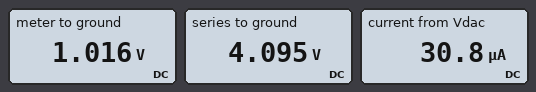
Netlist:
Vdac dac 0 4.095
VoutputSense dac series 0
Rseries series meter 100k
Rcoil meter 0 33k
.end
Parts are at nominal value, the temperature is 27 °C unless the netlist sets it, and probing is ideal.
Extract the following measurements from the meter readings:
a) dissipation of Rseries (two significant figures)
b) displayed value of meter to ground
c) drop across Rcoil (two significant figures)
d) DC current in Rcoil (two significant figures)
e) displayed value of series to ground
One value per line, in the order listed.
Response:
95 µW
1.016 V
1.0 V
31 µA
4.095 V
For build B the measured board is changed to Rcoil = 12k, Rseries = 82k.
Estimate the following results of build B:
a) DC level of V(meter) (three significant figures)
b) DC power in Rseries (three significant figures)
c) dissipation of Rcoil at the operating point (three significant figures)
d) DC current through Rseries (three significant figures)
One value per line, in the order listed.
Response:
523 mV
156 µW
22.8 µW
43.6 µA
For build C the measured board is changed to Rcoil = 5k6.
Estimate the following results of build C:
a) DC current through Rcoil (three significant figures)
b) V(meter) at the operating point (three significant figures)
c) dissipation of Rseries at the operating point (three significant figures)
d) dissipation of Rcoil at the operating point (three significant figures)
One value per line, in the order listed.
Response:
38.8 µA
217 mV
150 µW
8.42 µW
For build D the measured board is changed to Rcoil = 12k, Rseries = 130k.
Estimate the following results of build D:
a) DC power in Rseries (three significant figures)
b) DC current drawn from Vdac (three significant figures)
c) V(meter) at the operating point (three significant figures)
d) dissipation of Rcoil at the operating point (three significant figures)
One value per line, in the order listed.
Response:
108 µW
28.8 µA
346 mV
9.98 µW
